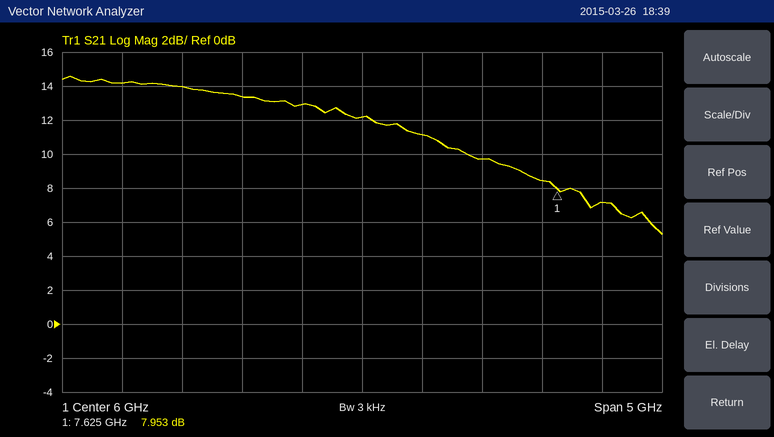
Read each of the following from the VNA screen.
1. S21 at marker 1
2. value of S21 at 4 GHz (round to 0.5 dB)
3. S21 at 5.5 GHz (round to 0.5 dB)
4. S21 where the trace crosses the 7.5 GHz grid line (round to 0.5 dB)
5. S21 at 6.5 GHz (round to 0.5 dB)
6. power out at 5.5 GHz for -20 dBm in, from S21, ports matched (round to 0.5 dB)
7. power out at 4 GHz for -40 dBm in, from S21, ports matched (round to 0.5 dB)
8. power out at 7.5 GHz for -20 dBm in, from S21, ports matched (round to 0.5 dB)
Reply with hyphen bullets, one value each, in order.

- 7.953 dB
- 14.0 dB
- 13.0 dB
- 8.5 dB
- 11.0 dB
- -7.0 dBm
- -26.0 dBm
- -11.5 dBm
